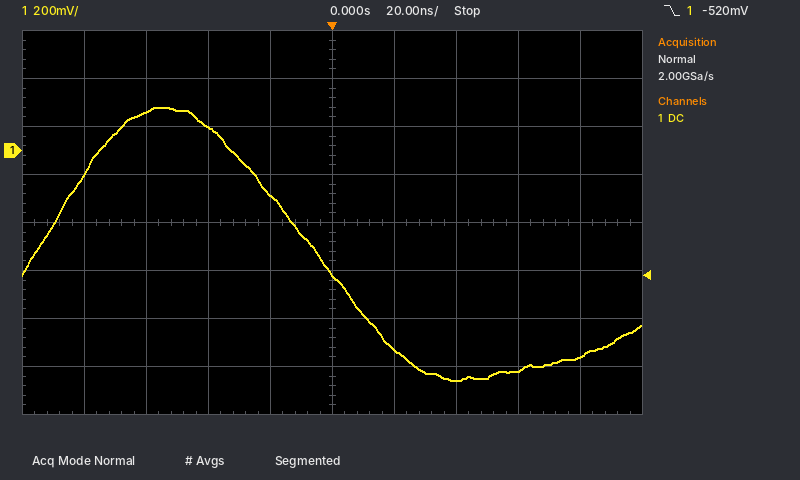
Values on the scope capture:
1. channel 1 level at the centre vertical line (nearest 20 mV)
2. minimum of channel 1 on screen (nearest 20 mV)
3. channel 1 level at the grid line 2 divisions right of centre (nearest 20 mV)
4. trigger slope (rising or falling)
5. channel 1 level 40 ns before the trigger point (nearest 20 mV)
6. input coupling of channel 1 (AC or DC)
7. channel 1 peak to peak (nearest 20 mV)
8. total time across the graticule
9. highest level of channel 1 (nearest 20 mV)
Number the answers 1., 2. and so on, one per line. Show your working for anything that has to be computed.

1. -520 mV
2. -960 mV
3. -960 mV
4. falling
5. 100 mV
6. DC
7. 180 mV − (-960 mV) = 1.14 V
8. 200 ns
9. 180 mV
